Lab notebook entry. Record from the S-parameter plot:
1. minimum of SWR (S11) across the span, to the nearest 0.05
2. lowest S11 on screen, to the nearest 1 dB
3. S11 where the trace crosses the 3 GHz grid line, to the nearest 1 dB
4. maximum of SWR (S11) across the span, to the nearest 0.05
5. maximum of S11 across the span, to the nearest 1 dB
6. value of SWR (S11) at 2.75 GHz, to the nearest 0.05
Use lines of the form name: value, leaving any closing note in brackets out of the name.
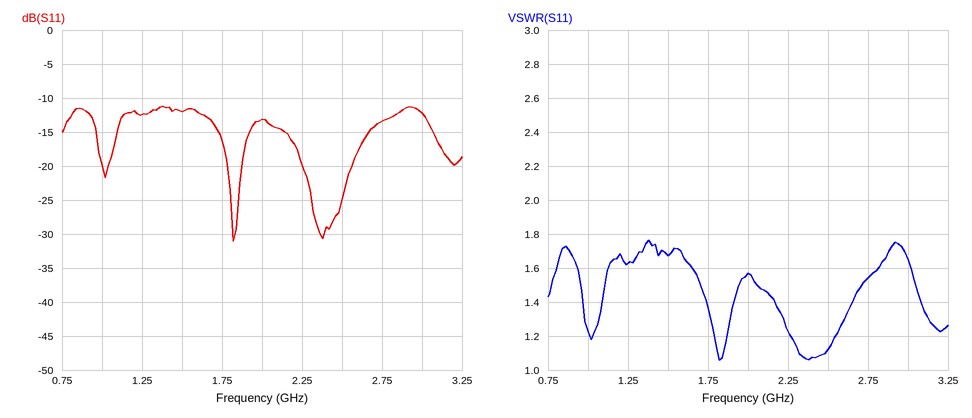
minimum of SWR (S11) across the span, to the nearest 0.05: 1.05
lowest S11 on screen, to the nearest 1 dB: -31 dB
S11 where the trace crosses the 3 GHz grid line, to the nearest 1 dB: -12 dB
maximum of SWR (S11) across the span, to the nearest 0.05: 1.75
maximum of S11 across the span, to the nearest 1 dB: -11 dB
value of SWR (S11) at 2.75 GHz, to the nearest 0.05: 1.55
